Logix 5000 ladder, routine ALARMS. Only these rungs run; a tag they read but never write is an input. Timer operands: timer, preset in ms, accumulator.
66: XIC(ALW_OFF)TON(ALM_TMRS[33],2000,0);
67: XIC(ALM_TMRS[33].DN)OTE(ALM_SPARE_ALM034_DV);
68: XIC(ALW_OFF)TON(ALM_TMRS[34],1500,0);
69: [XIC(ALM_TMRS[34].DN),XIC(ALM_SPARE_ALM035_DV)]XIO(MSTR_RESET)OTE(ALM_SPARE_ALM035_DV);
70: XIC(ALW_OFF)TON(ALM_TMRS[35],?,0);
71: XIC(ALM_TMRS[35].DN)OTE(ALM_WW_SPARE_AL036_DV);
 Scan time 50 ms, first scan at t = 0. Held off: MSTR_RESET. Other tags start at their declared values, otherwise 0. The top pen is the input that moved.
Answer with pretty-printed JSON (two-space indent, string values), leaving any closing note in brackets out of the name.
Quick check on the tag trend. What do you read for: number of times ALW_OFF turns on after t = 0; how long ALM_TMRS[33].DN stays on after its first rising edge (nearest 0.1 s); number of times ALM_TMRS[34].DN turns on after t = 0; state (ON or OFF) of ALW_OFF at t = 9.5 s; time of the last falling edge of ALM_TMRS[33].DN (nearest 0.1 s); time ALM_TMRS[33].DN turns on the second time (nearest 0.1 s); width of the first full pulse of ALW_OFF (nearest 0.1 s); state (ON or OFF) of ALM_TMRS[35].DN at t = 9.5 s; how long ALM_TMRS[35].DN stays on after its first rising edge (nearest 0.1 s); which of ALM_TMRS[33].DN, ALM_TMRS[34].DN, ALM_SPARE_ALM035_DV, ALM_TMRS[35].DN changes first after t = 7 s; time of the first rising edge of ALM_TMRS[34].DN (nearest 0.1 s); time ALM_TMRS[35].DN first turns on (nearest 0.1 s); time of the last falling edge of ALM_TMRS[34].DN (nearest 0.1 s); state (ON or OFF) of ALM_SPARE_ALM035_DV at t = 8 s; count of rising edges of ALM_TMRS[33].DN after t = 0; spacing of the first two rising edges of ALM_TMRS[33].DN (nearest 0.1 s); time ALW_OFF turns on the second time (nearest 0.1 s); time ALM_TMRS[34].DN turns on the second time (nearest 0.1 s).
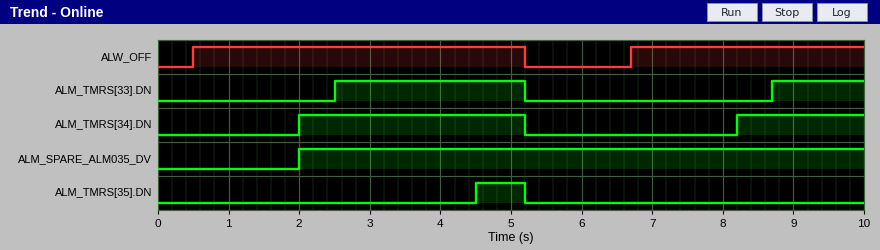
{
  "number of times ALW_OFF turns on after t = 0": "2",
  "how long ALM_TMRS[33].DN stays on after its first rising edge": "2.7 s",
  "number of times ALM_TMRS[34].DN turns on after t = 0": "2",
  "state (ON or OFF) of ALW_OFF at t = 9.5 s": "ON",
  "time of the last falling edge of ALM_TMRS[33].DN": "5.2 s",
  "time ALM_TMRS[33].DN turns on the second time": "8.7 s",
  "width of the first full pulse of ALW_OFF": "4.7 s",
  "state (ON or OFF) of ALM_TMRS[35].DN at t = 9.5 s": "OFF",
  "how long ALM_TMRS[35].DN stays on after its first rising edge": "0.7 s",
  "which of ALM_TMRS[33].DN, ALM_TMRS[34].DN, ALM_SPARE_ALM035_DV, ALM_TMRS[35].DN changes first after t = 7 s": "ALM_TMRS[34].DN",
  "time of the first rising edge of ALM_TMRS[34].DN": "2.0 s",
  "time ALM_TMRS[35].DN first turns on": "4.5 s",
  "time of the last falling edge of ALM_TMRS[34].DN": "5.2 s",
  "state (ON or OFF) of ALM_SPARE_ALM035_DV at t = 8 s": "ON",
  "count of rising edges of ALM_TMRS[33].DN after t = 0": "2",
  "spacing of the first two rising edges of ALM_TMRS[33].DN": "6.2 s",
  "time ALW_OFF turns on the second time": "6.7 s",
  "time ALM_TMRS[34].DN turns on the second time": "8.2 s"
}
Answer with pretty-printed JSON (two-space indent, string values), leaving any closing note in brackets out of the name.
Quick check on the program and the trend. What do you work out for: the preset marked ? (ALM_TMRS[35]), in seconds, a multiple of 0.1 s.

{
  "the preset marked ? (ALM_TMRS[35]), in seconds, a multiple of 0.1 s": "4.0 s"
}
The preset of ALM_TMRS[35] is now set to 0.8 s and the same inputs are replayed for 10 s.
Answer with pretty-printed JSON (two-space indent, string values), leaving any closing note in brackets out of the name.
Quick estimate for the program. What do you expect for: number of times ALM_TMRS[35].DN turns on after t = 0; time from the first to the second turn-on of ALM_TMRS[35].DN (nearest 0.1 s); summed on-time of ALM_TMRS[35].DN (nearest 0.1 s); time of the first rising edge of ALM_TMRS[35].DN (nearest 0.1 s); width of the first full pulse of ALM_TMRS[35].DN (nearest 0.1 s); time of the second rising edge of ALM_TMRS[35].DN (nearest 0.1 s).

{
  "number of times ALM_TMRS[35].DN turns on after t = 0": "2",
  "time from the first to the second turn-on of ALM_TMRS[35].DN": "6.2 s",
  "summed on-time of ALM_TMRS[35].DN": "6.4 s",
  "time of the first rising edge of ALM_TMRS[35].DN": "1.3 s",
  "width of the first full pulse of ALM_TMRS[35].DN": "3.9 s",
  "time of the second rising edge of ALM_TMRS[35].DN": "7.5 s"
}
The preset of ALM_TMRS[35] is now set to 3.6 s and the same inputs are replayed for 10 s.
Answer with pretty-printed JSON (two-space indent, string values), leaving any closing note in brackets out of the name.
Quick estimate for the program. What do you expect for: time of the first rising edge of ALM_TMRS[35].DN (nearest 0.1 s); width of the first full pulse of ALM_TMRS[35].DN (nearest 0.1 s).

{
  "time of the first rising edge of ALM_TMRS[35].DN": "4.1 s",
  "width of the first full pulse of ALM_TMRS[35].DN": "1.1 s"
}
